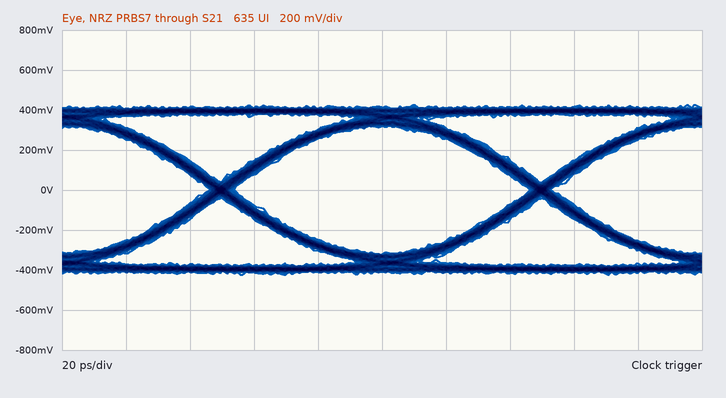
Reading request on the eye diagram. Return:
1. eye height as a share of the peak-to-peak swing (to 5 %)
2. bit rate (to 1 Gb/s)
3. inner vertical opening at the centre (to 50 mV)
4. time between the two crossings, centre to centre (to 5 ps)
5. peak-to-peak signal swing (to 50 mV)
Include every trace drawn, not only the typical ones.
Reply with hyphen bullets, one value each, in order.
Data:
- 75 %
- 10 Gb/s
- 650 mV
- 100 ps
- 850 mV
